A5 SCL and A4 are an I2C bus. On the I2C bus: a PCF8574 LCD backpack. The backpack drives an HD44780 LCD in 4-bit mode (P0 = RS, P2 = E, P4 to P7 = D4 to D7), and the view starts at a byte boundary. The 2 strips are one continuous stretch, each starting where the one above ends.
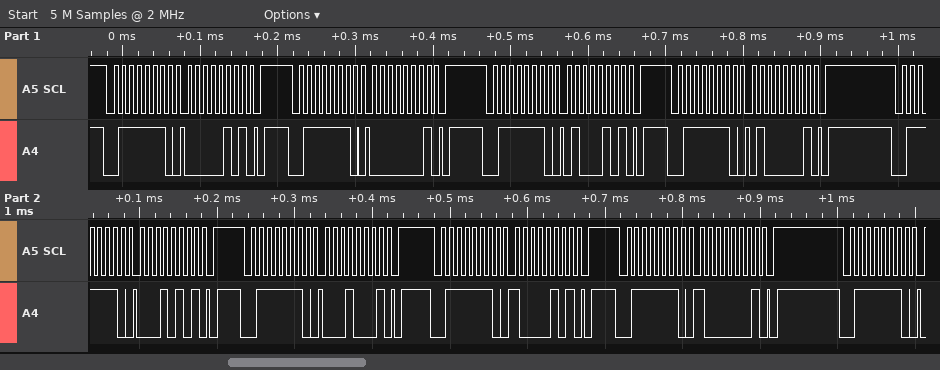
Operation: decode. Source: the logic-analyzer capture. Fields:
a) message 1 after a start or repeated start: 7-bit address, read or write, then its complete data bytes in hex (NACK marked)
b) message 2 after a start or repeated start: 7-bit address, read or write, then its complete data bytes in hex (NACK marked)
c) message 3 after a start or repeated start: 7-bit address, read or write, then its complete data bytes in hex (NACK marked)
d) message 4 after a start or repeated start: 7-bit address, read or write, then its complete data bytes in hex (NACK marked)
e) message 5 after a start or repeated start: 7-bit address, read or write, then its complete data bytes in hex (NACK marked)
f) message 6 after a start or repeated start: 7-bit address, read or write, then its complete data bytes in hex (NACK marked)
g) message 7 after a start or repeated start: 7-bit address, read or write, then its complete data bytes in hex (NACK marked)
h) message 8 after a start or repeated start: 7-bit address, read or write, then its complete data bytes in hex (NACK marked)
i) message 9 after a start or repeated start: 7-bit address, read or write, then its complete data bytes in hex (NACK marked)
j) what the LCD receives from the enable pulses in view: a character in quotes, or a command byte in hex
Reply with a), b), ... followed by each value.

a) 0x3F write: 05
b) 0x3F write: 01
c) 0x3F write: 45
d) 0x3F write: 41
e) 0x3F write: 15
f) 0x3F write: 11
g) 0x3F write: 85
h) 0x3F write: 81
i) 0x3F write
j) data 0x04 data 0x18
